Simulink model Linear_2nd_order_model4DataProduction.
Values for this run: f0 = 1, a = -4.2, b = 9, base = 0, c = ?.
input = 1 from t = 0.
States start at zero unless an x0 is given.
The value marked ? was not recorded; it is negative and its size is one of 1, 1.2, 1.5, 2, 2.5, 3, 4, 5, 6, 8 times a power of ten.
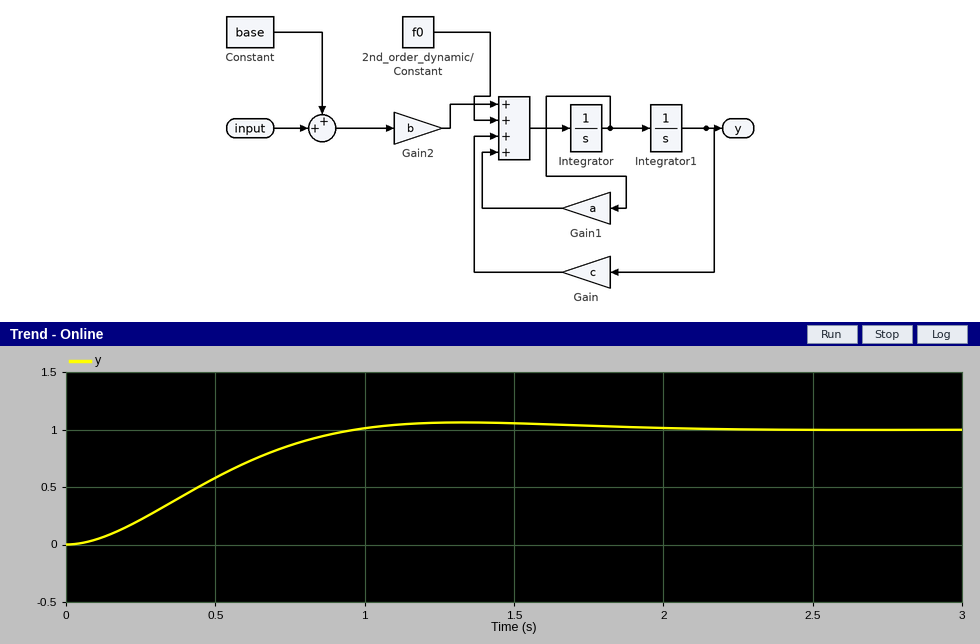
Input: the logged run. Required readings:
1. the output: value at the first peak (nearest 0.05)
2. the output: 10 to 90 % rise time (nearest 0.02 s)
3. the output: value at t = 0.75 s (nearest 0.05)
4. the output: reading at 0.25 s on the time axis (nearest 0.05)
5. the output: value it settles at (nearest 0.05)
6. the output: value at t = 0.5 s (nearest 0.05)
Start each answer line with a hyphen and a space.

- 1.05
- 0.64 s
- 0.85
- 0.20
- 1.00
- 0.60
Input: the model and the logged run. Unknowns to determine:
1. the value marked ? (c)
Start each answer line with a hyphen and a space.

- -10
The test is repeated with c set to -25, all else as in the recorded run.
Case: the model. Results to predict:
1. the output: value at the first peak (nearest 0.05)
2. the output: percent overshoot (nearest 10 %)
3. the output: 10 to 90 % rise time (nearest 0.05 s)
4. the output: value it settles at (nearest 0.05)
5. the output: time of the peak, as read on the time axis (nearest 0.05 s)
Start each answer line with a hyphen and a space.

- 0.50
- 20 %
- 0.30 s
- 0.40
- 0.70 s
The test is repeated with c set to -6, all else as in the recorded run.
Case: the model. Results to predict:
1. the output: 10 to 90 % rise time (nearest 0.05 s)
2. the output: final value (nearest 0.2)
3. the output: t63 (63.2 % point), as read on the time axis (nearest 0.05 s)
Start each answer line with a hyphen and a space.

- 1.10 s
- 1.6
- 0.80 s
